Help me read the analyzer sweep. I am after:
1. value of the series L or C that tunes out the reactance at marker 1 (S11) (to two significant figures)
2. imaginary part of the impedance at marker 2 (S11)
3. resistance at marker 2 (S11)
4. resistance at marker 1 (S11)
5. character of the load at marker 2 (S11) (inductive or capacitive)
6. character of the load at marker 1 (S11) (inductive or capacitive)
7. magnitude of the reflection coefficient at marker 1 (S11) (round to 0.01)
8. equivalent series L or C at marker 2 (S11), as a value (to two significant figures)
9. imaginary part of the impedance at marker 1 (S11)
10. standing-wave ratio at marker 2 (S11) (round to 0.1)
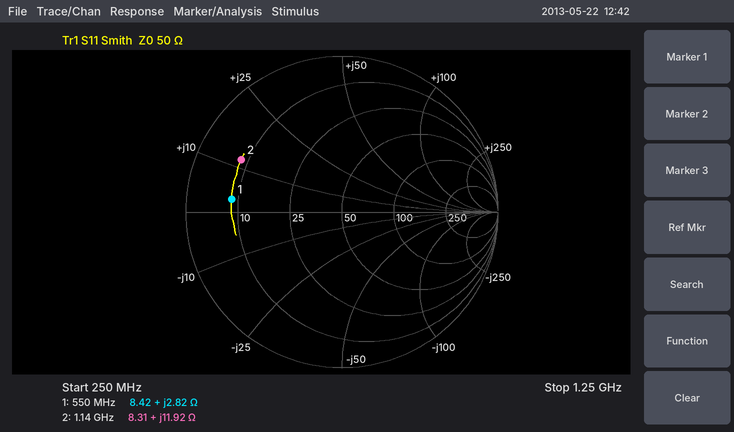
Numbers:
100 pF
+11.92 Ω
8.31 Ω
8.42 Ω
inductive
inductive
0.71
1.7 nH
+2.82 Ω
6.4
